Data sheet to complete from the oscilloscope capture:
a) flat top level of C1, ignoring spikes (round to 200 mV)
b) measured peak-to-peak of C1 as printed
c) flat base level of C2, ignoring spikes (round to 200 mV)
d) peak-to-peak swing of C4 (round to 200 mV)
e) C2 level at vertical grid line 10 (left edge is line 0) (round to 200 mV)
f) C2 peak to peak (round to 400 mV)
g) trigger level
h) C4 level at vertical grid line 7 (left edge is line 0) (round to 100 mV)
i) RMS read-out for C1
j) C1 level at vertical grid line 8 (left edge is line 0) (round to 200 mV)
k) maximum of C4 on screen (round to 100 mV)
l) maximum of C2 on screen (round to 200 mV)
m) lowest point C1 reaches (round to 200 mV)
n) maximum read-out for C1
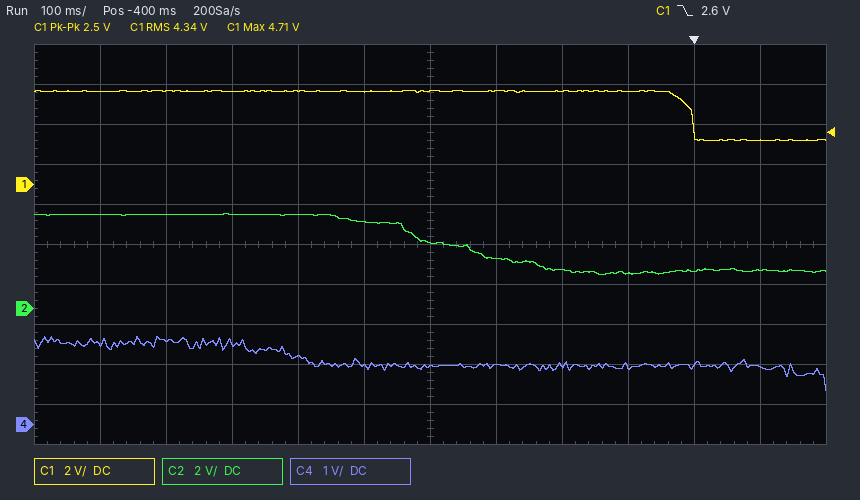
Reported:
4.6 V
2.5 V
1.8 V
1.4 V
1.8 V
3.2 V
2.6 V
1.5 V
4.34 V
4.6 V
2.2 V
4.8 V
2.2 V
4.71 V
